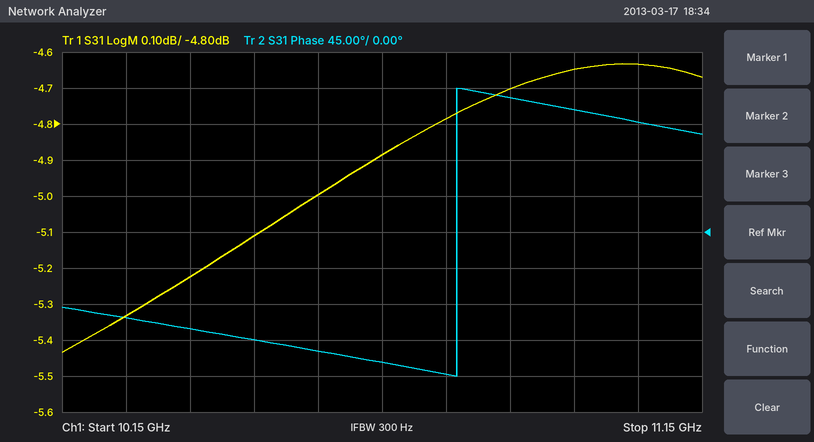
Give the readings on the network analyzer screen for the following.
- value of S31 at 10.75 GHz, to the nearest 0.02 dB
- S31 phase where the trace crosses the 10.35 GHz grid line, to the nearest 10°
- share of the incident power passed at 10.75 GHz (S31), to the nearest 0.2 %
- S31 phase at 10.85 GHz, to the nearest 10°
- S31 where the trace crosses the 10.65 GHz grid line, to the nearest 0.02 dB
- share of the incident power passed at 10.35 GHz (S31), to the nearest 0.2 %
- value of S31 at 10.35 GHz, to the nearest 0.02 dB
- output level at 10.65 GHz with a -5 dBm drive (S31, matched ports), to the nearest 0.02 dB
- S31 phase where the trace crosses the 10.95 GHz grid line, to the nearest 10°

-4.78 dB
-120°
33.2 %
170°
-4.88 dB
30.0 %
-5.22 dB
-9.88 dBm
150°
